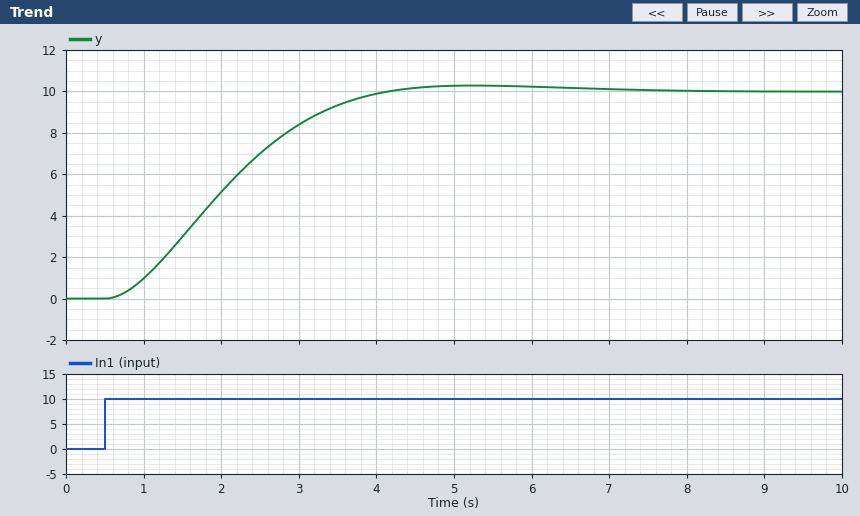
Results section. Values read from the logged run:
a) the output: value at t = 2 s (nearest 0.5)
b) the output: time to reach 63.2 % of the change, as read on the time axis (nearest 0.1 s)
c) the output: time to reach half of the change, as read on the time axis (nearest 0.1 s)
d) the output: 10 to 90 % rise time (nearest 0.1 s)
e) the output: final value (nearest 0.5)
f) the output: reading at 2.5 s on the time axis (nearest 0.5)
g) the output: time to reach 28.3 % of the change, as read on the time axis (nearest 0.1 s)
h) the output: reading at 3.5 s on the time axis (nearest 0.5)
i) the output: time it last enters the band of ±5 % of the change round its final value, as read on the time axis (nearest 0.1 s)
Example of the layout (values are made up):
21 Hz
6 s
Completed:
5.0
2.3 s
2.0 s
2.3 s
10.0
7.0
1.5 s
9.5
3.6 s
